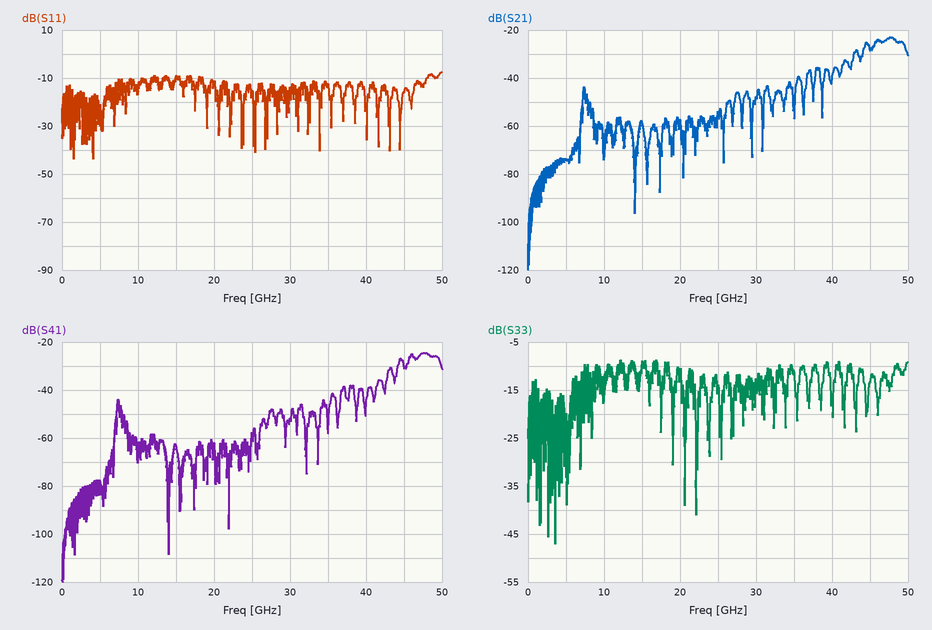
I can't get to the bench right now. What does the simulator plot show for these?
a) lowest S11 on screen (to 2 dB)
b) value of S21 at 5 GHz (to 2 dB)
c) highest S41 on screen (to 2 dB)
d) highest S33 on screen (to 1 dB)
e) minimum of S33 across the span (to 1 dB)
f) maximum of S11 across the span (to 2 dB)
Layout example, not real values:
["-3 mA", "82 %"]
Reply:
["-44 dB", "-74 dB", "-24 dB", "-9 dB", "-47 dB", "-8 dB"]
